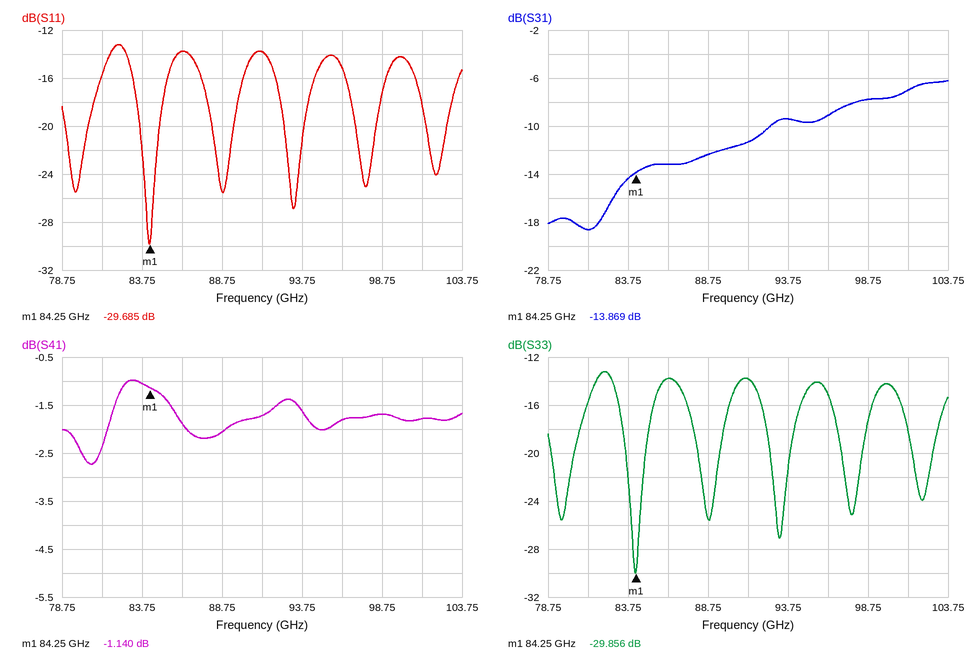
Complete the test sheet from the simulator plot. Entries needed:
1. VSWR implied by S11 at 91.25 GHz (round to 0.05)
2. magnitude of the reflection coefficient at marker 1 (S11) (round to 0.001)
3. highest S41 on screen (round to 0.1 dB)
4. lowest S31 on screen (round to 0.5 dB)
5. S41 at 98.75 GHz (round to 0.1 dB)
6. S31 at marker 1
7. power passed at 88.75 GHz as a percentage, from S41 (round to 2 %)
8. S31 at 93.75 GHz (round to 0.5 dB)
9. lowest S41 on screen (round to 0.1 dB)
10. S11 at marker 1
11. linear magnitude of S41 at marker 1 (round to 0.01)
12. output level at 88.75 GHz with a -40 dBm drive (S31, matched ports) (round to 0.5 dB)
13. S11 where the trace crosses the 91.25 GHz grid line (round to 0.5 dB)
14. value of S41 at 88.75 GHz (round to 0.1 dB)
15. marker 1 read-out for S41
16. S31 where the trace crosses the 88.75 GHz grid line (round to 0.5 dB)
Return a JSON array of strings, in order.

["1.50", "0.033", "-1.0 dB", "-18.5 dB", "-1.7 dB", "-13.869 dB", "62 %", "-9.5 dB", "-2.7 dB", "-29.685 dB", "0.88", "-52.5 dBm", "-14.0 dB", "-2.1 dB", "-1.140 dB", "-12.5 dB"]
